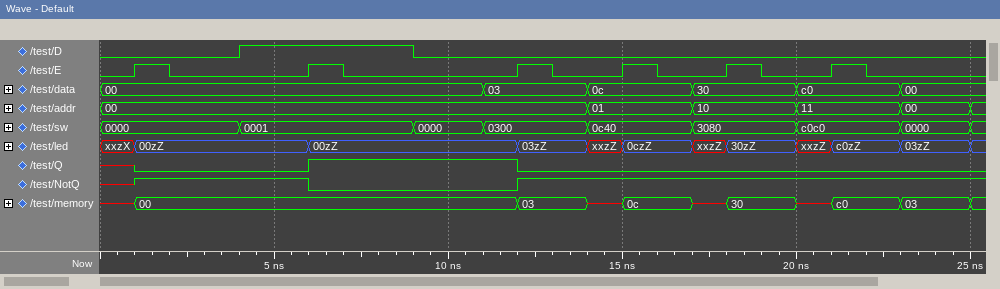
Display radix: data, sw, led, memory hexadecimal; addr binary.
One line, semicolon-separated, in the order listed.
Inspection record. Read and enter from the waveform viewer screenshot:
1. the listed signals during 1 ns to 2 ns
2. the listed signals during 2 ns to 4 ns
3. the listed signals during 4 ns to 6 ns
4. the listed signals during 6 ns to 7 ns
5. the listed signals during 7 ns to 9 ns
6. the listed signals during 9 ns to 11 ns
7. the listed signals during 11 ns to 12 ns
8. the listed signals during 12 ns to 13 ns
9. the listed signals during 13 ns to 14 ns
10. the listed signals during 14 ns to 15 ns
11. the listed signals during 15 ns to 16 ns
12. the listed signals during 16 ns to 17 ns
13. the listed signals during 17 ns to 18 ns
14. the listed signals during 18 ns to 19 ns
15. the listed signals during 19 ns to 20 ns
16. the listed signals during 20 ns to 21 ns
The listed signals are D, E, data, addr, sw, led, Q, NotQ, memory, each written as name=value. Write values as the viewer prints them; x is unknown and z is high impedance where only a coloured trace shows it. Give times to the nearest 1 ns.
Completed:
D=0, E=1, data=00, addr=00, sw=0000, led=00zZ, Q=0, NotQ=1, memory=00; D=0, E=0, data=00, addr=00, sw=0000, led=00zZ, Q=0, NotQ=1, memory=00; D=1, E=0, data=00, addr=00, sw=0001, led=00zZ, Q=0, NotQ=1, memory=00; D=1, E=1, data=00, addr=00, sw=0001, led=00zZ, Q=1, NotQ=0, memory=00; D=1, E=0, data=00, addr=00, sw=0001, led=00zZ, Q=1, NotQ=0, memory=00; D=0, E=0, data=00, addr=00, sw=0000, led=00zZ, Q=1, NotQ=0, memory=00; D=0, E=0, data=03, addr=00, sw=0300, led=00zZ, Q=1, NotQ=0, memory=00; D=0, E=1, data=03, addr=00, sw=0300, led=03zZ, Q=0, NotQ=1, memory=03; D=0, E=0, data=03, addr=00, sw=0300, led=03zZ, Q=0, NotQ=1, memory=03; D=0, E=0, data=0c, addr=01, sw=0c40, led=xxzZ, Q=0, NotQ=1, memory=x; D=0, E=1, data=0c, addr=01, sw=0c40, led=0czZ, Q=0, NotQ=1, memory=0c; D=0, E=0, data=0c, addr=01, sw=0c40, led=0czZ, Q=0, NotQ=1, memory=0c; D=0, E=0, data=30, addr=10, sw=3080, led=xxzZ, Q=0, NotQ=1, memory=x; D=0, E=1, data=30, addr=10, sw=3080, led=30zZ, Q=0, NotQ=1, memory=30; D=0, E=0, data=30, addr=10, sw=3080, led=30zZ, Q=0, NotQ=1, memory=30; D=0, E=0, data=c0, addr=11, sw=c0c0, led=xxzZ, Q=0, NotQ=1, memory=x
